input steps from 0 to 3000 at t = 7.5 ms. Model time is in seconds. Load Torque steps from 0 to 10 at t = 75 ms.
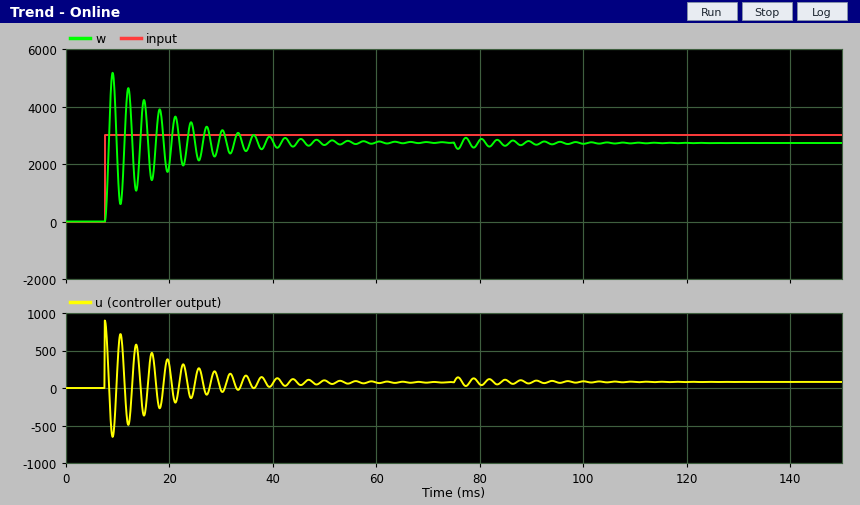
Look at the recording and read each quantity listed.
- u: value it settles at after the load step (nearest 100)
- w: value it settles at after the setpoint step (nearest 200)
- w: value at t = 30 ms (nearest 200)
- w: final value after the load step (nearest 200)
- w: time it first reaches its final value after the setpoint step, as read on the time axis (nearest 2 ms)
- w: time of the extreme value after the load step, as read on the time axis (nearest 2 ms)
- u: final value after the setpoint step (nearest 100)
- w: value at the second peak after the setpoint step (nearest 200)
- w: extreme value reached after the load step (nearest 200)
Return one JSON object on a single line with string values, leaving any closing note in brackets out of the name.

{"u: value it settles at after the load step": "100", "w: value it settles at after the setpoint step": "2800", "w: value at t = 30 ms": "3200", "w: final value after the load step": "2800", "w: time it first reaches its final value after the setpoint step, as read on the time axis": "8 ms", "w: time of the extreme value after the load step, as read on the time axis": "76 ms", "u: final value after the setpoint step": "100", "w: value at the second peak after the setpoint step": "4600", "w: extreme value reached after the load step": "2600"}
